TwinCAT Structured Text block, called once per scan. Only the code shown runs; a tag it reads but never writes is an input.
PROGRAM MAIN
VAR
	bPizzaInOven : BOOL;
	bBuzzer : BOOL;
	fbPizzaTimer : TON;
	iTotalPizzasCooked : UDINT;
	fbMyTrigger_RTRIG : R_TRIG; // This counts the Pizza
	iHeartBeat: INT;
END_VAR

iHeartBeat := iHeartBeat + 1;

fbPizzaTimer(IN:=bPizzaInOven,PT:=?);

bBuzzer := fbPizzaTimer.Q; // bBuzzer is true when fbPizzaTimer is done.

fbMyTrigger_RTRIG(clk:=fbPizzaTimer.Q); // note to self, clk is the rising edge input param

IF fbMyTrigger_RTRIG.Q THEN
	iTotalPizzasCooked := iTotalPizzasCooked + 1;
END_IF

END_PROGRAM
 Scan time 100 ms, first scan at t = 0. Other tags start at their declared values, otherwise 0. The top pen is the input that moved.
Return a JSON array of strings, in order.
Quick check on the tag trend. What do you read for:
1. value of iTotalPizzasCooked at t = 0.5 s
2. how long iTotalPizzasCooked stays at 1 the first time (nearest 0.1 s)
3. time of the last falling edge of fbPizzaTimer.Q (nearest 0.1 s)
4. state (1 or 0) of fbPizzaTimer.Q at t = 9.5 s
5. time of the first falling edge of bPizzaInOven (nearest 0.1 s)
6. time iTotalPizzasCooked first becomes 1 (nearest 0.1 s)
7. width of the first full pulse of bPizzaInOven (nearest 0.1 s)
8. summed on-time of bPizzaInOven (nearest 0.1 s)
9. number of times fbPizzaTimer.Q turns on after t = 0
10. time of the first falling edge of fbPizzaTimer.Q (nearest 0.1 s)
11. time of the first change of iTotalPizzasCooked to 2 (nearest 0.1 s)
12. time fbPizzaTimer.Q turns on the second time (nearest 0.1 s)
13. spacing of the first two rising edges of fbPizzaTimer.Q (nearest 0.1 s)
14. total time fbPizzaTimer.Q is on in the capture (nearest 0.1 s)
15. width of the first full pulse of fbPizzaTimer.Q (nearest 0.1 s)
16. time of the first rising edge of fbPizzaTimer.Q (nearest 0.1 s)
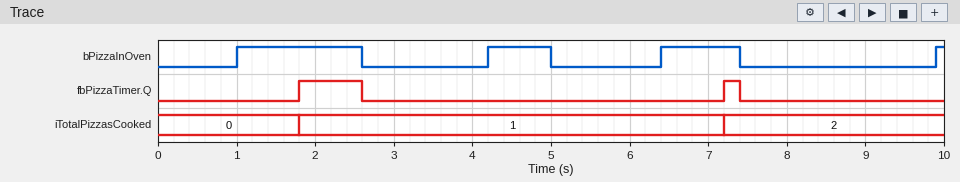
["0", "5.4 s", "7.4 s", "0", "2.6 s", "1.8 s", "1.6 s", "3.5 s", "2", "2.6 s", "7.2 s", "7.2 s", "5.4 s", "1.0 s", "0.8 s", "1.8 s"]
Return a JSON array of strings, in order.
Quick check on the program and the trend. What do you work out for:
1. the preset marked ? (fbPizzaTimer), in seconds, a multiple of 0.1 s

["0.8 s"]
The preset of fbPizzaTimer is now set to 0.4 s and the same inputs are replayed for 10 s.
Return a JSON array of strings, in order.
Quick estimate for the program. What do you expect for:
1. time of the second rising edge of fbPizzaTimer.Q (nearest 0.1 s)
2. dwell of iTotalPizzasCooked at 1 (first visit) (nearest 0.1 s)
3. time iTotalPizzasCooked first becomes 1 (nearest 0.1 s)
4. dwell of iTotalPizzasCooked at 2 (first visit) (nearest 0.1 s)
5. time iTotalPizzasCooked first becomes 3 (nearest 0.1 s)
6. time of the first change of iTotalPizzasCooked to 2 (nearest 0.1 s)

["4.6 s", "3.2 s", "1.4 s", "2.2 s", "6.8 s", "4.6 s"]
